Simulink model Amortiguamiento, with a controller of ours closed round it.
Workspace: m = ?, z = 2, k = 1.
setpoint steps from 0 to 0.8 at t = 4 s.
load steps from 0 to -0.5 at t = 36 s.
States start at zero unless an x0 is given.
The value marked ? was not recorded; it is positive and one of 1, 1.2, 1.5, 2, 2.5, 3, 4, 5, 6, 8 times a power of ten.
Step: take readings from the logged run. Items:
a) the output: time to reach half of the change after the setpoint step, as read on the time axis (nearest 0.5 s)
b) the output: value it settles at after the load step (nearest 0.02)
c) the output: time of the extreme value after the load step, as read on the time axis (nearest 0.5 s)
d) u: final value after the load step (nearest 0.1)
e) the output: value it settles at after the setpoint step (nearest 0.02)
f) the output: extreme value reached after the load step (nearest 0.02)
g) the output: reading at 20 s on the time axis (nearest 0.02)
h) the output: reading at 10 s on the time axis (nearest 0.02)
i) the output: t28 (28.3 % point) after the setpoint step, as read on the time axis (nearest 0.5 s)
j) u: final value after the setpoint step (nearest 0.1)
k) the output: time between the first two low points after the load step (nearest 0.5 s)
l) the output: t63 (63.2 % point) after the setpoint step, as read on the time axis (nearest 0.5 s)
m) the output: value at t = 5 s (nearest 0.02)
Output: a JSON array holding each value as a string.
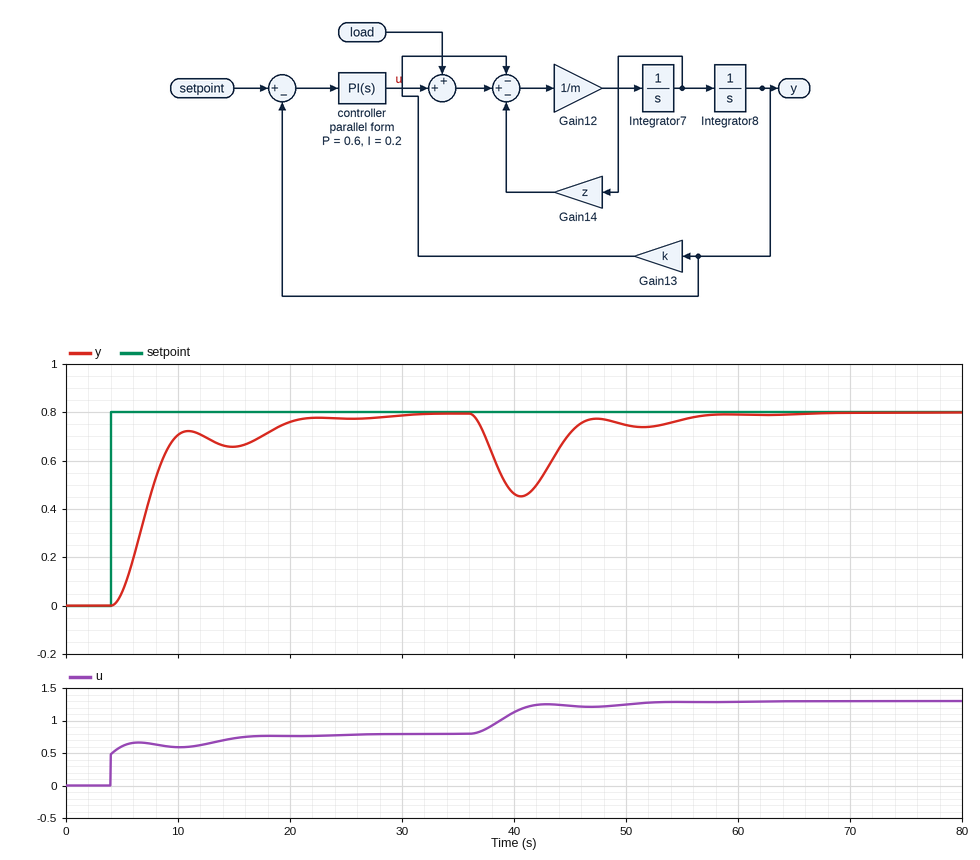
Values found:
["7.0 s", "0.80", "40.5 s", "1.3", "0.80", "0.46", "0.76", "0.70", "6.0 s", "0.8", "11.0 s", "8.0 s", "0.06"]
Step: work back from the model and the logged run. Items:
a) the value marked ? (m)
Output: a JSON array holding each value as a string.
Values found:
["4"]
